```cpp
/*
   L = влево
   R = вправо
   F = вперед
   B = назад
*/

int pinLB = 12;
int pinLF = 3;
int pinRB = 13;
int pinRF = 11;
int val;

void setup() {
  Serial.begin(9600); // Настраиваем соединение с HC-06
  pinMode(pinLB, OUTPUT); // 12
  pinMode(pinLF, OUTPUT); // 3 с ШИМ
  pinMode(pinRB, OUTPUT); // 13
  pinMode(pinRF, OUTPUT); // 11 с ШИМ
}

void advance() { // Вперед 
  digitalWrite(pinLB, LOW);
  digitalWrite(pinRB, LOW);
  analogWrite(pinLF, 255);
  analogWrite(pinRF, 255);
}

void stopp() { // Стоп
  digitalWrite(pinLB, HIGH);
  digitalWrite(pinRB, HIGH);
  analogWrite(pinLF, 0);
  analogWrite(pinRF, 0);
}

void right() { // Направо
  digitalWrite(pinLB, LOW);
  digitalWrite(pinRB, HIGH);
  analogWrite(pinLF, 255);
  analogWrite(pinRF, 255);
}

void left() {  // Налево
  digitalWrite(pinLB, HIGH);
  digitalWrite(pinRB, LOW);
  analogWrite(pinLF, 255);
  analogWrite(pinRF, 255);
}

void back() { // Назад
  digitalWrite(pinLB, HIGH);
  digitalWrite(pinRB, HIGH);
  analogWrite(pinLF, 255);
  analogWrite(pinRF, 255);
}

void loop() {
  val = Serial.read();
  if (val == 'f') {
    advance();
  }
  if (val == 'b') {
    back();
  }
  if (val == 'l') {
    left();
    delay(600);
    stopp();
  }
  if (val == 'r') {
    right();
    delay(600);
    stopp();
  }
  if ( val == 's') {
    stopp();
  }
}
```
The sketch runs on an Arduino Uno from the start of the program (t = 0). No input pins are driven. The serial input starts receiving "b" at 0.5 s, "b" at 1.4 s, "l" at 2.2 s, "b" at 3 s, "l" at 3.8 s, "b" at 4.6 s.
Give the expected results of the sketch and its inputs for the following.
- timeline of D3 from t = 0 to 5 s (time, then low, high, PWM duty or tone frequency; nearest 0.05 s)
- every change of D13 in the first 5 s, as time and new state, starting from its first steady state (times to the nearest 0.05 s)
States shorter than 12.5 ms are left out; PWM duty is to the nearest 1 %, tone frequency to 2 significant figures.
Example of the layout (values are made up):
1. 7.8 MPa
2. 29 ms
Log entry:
1. 0 s low; 0.5 s high; 2.8 s low; 3 s high; 4.4 s low; 4.6 s high
2. 0 s low; 0.5 s high; 2.2 s low; 2.8 s high; 3.8 s low; 4.4 s high
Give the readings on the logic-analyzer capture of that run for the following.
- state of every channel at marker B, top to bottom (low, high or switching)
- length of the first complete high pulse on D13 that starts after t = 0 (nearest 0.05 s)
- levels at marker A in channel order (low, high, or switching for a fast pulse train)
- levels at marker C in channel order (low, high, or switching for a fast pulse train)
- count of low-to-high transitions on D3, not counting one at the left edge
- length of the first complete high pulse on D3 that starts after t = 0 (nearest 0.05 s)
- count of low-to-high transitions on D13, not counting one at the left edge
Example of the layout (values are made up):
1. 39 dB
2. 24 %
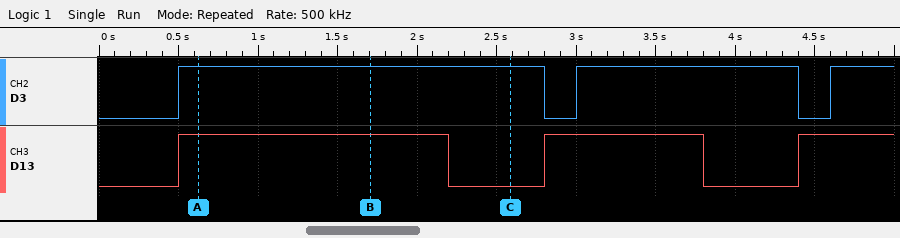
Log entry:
1. D3 high, D13 high
2. 1.70 s
3. D3 high, D13 high
4. D3 high, D13 low
5. 3
6. 2.30 s
7. 3
